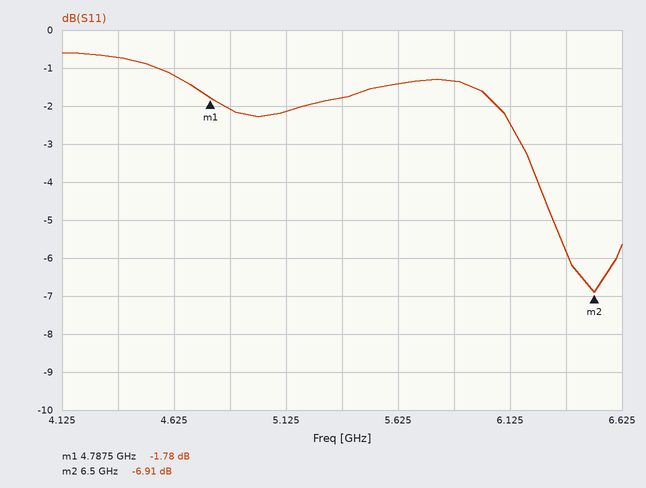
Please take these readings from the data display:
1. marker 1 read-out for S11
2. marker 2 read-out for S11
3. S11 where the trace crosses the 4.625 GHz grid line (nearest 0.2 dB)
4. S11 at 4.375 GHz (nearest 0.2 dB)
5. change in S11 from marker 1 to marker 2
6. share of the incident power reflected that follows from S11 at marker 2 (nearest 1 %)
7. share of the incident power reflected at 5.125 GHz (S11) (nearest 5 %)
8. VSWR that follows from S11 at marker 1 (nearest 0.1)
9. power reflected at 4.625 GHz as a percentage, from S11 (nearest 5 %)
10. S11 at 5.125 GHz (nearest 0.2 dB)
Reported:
-1.78 dB
-6.91 dB
-1.2 dB
-0.8 dB
-5.13 dB
20 %
60 %
9.8
75 %
-2.2 dB
